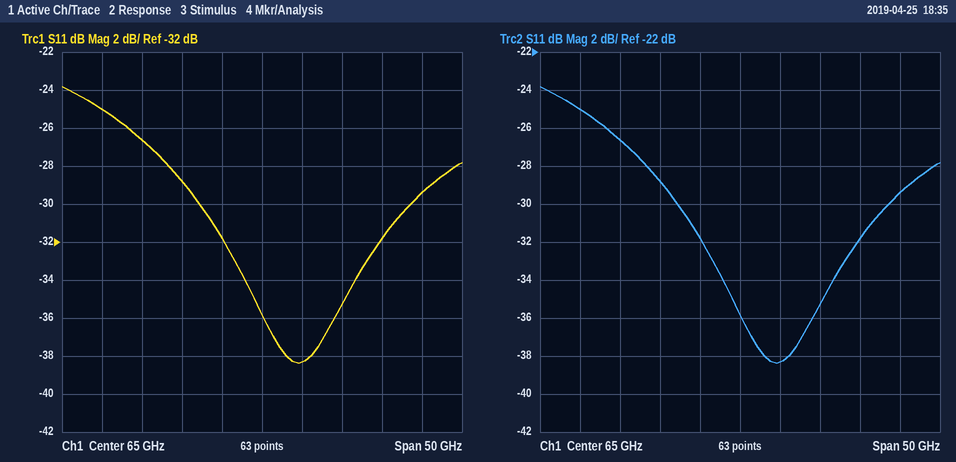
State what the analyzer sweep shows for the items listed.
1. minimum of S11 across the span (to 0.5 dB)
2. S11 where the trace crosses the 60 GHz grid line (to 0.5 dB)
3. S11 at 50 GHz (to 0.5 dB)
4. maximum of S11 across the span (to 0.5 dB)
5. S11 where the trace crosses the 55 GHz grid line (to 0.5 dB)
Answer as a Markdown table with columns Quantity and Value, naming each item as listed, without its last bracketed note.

| Quantity | Value |
|---|---|
| minimum of S11 across the span | -38.5 dB |
| S11 where the trace crosses the 60 GHz grid line | -32.0 dB |
| S11 at 50 GHz | -26.5 dB |
| maximum of S11 across the span | -24.0 dB |
| S11 where the trace crosses the 55 GHz grid line | -29.0 dB |
